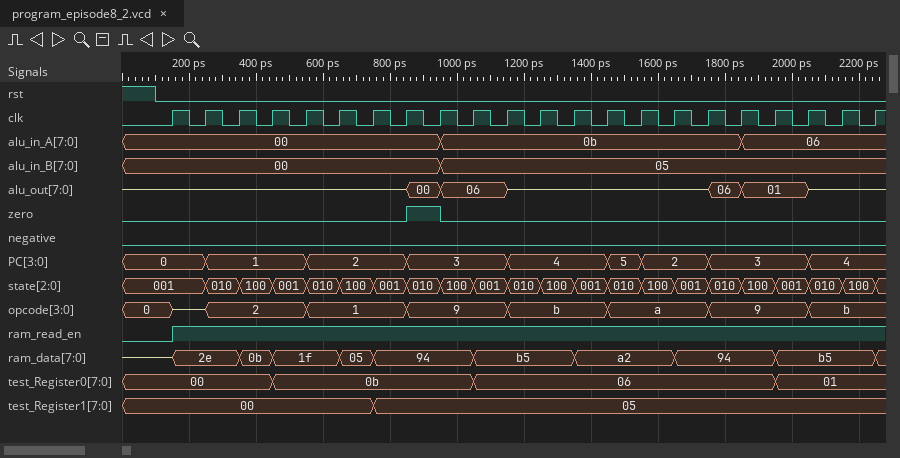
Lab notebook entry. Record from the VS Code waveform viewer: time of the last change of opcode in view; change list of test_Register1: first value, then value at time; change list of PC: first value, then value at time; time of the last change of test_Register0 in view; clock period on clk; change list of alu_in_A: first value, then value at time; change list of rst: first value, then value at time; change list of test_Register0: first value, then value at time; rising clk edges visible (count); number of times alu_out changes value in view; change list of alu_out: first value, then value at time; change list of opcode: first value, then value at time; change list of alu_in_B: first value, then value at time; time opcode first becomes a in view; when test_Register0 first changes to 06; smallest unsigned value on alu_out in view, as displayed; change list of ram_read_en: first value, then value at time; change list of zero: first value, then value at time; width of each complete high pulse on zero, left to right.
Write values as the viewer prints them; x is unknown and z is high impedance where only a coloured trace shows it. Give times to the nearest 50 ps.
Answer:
2050 ps
00, 05 at 750 ps
0, 1 at 250 ps, 2 at 550 ps, 3 at 850 ps, 4 at 1150 ps, 5 at 1450 ps, 2 at 1550 ps, 3 at 1750 ps, 4 at 2050 ps
1950 ps
100 ps
00, 0b at 950 ps, 06 at 1850 ps
1, 0 at 100 ps
00, 0b at 450 ps, 06 at 1050 ps, 01 at 1950 ps
22
6
z, 00 at 850 ps, 06 at 950 ps, z at 1150 ps, 06 at 1750 ps, 01 at 1850 ps, z at 2050 ps
0, z at 150 ps, 2 at 250 ps, 1 at 550 ps, 9 at 850 ps, b at 1150 ps, a at 1450 ps, 9 at 1750 ps, b at 2050 ps
00, 05 at 950 ps
1450 ps
1050 ps
00
0, 1 at 150 ps
0, 1 at 850 ps, 0 at 950 ps
100 ps
